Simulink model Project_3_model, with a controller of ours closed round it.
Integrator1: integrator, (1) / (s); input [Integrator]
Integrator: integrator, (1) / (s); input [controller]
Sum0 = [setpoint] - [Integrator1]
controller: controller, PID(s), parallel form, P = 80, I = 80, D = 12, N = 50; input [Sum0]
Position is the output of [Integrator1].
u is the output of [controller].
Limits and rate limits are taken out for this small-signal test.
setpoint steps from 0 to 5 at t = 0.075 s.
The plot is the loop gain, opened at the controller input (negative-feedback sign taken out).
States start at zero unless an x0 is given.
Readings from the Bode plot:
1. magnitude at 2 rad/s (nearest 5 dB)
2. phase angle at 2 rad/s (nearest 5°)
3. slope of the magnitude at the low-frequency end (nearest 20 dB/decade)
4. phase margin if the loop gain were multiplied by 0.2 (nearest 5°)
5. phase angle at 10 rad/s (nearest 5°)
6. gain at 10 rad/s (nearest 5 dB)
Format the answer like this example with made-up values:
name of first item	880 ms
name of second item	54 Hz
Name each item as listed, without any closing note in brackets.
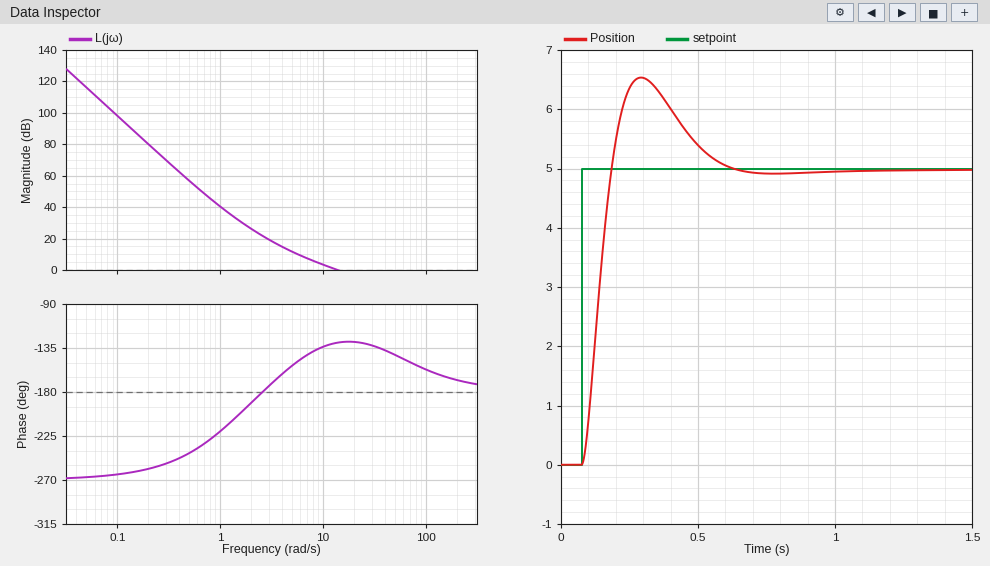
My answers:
magnitude at 2 rad/s	25 dB
phase angle at 2 rad/s	-190°
slope of the magnitude at the low-frequency end	-60 dB/decade
phase margin if the loop gain were multiplied by 0.2	20°
phase angle at 10 rad/s	-135°
gain at 10 rad/s	5 dB
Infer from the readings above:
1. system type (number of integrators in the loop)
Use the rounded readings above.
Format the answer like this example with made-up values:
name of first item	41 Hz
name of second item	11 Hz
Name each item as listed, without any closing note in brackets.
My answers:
system type	3
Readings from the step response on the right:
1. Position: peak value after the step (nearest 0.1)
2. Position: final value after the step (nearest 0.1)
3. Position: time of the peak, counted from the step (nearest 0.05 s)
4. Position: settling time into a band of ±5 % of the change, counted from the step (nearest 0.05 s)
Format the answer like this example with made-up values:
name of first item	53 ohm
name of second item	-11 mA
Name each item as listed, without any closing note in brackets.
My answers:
Position: peak value after the step	6.5
Position: final value after the step	5.0
Position: time of the peak, counted from the step	0.20 s
Position: settling time into a band of ±5 % of the change, counted from the step	0.45 s
